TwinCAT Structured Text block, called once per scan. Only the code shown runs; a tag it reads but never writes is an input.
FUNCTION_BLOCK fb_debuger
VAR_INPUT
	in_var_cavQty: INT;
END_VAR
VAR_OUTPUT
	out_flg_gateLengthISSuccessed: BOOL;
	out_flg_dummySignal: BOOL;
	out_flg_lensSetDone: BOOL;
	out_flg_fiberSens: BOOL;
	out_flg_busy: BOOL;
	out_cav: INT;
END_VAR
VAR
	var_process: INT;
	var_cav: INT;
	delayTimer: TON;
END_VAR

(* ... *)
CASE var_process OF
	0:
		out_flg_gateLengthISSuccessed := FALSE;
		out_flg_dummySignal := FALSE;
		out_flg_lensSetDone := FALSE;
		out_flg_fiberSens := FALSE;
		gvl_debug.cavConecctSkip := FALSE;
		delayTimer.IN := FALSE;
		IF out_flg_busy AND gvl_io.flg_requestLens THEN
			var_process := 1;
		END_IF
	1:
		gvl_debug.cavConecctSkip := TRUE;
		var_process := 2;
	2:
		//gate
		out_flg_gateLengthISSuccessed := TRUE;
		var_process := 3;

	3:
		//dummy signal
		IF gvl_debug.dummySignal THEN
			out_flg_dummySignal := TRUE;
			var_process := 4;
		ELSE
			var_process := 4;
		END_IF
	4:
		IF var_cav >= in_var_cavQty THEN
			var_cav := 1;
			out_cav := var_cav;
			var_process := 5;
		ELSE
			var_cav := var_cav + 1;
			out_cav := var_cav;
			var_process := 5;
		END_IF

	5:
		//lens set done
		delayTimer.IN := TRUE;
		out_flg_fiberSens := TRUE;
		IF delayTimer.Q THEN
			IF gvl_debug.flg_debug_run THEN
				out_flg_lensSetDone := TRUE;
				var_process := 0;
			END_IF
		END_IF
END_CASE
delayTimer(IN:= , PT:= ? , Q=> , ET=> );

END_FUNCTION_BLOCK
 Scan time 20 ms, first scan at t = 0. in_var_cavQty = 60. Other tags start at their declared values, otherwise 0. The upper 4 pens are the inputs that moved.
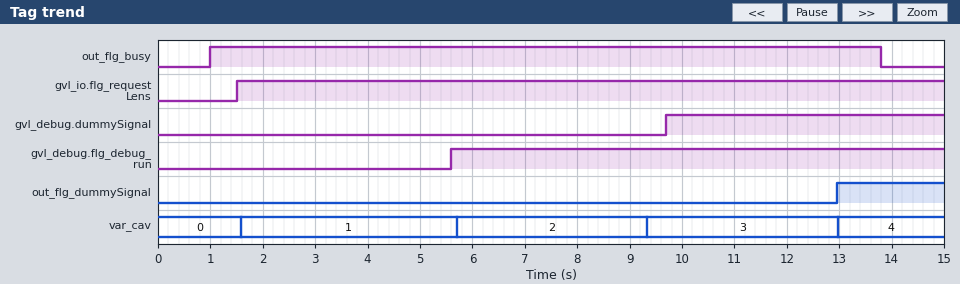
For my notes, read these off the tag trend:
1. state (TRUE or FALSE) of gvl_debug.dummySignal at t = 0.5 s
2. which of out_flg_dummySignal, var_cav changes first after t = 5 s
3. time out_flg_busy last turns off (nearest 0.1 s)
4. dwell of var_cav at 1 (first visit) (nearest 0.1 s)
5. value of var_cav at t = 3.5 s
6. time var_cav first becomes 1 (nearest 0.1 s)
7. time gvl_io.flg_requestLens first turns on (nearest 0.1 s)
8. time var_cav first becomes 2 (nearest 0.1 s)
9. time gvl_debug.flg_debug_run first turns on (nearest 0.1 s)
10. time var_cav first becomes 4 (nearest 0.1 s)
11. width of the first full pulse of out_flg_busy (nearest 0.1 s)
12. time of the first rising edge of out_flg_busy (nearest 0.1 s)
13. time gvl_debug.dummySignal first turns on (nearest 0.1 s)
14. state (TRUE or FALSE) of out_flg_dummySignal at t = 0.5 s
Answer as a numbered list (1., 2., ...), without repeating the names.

1. FALSE
2. var_cav
3. 13.8 s
4. 4.1 s
5. 1
6. 1.6 s
7. 1.5 s
8. 5.7 s
9. 5.6 s
10. 13.0 s
11. 12.8 s
12. 1.0 s
13. 9.7 s
14. FALSE
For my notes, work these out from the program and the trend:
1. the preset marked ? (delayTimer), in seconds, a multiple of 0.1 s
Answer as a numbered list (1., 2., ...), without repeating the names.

1. 3.5 s
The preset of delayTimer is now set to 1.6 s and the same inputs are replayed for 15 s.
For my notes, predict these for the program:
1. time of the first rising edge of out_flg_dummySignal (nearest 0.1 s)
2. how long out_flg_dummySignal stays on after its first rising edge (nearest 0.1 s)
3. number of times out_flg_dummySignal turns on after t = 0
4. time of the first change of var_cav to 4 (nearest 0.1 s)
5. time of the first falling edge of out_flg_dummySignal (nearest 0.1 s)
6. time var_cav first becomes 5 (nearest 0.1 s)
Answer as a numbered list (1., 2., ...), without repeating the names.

1. 10.9 s
2. 1.7 s
3. 2
4. 9.2 s
5. 12.6 s
6. 10.9 s
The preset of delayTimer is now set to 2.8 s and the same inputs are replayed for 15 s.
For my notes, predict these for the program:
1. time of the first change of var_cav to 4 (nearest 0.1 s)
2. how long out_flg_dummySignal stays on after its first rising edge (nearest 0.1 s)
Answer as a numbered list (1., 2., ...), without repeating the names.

1. 11.6 s
2. 2.9 s
